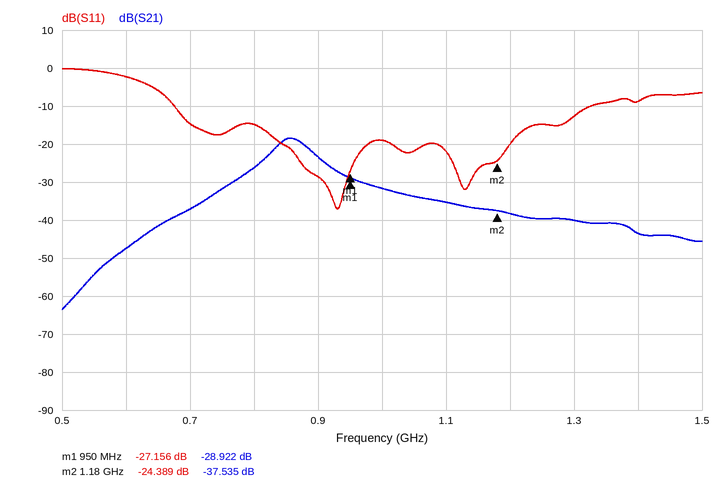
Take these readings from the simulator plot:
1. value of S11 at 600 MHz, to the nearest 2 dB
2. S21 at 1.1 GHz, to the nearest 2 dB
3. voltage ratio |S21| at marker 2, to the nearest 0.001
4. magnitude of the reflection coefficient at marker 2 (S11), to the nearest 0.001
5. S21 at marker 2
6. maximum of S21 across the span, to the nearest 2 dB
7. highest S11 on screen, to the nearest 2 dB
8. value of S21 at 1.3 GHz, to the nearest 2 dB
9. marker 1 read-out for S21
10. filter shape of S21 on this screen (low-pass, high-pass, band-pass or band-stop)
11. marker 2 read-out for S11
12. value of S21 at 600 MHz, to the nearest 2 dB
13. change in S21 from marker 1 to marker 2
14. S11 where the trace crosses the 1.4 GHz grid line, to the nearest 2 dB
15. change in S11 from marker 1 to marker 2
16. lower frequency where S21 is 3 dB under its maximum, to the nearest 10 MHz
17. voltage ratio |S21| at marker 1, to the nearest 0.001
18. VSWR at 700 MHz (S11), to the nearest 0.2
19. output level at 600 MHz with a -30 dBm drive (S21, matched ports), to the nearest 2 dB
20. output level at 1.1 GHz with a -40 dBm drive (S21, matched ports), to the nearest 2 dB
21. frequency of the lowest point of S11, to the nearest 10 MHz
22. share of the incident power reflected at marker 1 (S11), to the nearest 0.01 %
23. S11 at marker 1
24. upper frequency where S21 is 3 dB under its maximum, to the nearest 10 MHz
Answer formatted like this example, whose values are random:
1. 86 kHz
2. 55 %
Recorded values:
1. -2 dB
2. -36 dB
3. 0.013
4. 0.060
5. -37.535 dB
6. -18 dB
7. 0 dB
8. -40 dB
9. -28.922 dB
10. band-pass
11. -24.389 dB
12. -48 dB
13. -8.613 dB
14. -8 dB
15. 2.767 dB
16. 830 MHz
17. 0.036
18. 1.4
19. -78 dBm
20. -76 dBm
21. 930 MHz
22. 0.19 %
23. -27.156 dB
24. 890 MHz
